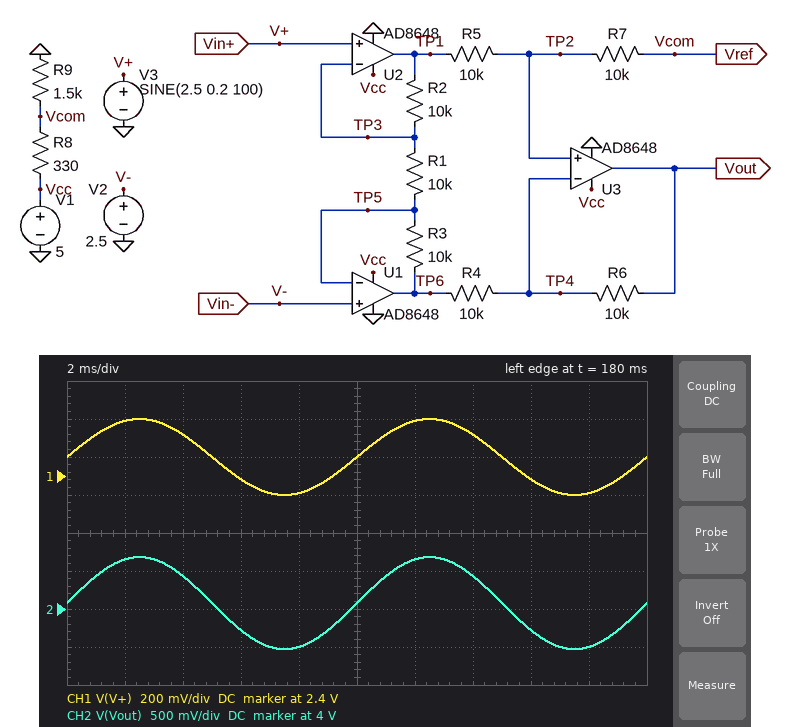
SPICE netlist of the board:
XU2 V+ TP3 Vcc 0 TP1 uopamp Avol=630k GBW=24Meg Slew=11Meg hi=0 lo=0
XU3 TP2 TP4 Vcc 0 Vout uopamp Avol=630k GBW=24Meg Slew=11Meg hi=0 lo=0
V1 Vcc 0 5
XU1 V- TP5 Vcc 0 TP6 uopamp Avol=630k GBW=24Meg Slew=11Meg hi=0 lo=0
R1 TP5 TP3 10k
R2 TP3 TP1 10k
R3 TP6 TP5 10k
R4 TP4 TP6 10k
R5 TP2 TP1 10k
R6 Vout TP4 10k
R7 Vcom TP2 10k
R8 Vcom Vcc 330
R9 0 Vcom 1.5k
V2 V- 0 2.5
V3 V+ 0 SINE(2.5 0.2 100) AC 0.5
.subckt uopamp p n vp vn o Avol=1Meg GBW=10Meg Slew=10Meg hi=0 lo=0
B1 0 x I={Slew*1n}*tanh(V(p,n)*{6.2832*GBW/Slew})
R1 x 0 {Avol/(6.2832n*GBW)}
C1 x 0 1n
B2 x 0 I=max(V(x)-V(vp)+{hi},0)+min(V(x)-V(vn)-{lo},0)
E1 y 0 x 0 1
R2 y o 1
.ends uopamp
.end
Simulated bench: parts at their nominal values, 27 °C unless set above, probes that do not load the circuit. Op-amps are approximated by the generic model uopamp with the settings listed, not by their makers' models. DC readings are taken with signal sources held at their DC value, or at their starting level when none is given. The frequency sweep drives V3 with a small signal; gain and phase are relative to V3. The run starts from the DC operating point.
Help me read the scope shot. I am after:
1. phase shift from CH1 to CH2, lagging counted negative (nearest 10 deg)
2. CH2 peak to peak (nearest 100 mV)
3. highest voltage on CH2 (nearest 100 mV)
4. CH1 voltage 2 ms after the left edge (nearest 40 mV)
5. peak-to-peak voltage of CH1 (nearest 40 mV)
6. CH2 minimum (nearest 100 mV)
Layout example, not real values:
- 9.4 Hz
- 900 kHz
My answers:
- 0 deg
- 1.2 V
- 4.7 V
- 2.68 V
- 400 mV
- 3.5 V
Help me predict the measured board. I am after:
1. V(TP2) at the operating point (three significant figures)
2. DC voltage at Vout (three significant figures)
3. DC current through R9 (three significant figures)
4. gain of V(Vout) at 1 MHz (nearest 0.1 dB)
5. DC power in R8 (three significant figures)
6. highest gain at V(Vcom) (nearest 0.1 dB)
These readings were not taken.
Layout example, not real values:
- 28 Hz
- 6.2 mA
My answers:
- 3.29 V
- 4.08 V
- 2.72 mA
- 9.5 dB
- 2.58 mW
- -31.5 dB
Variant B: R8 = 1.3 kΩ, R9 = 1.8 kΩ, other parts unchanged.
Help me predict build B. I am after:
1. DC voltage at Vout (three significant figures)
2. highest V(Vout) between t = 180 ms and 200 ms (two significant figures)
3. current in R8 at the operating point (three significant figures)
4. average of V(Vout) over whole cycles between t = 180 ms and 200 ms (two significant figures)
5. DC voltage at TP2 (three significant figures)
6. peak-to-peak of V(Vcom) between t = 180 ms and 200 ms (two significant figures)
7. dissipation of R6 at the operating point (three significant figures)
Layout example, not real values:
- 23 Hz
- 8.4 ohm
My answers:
- 2.89 V
- 3.5 V
- 1.62 mA
- 2.9 V
- 2.69 V
- 29 mV
- 3.77 µW
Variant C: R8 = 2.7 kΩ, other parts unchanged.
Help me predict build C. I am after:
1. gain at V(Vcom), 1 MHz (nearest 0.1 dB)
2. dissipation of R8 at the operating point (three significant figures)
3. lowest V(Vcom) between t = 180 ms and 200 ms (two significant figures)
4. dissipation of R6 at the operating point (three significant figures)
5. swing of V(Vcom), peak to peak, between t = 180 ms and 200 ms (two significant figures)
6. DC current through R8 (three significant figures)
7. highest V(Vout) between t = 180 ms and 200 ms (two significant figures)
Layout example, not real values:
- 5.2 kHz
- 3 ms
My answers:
- -20.8 dB
- 3.75 mW
- 1.8 V
- 11.6 µW
- 37 mV
- 1.18 mA
- 2.4 V
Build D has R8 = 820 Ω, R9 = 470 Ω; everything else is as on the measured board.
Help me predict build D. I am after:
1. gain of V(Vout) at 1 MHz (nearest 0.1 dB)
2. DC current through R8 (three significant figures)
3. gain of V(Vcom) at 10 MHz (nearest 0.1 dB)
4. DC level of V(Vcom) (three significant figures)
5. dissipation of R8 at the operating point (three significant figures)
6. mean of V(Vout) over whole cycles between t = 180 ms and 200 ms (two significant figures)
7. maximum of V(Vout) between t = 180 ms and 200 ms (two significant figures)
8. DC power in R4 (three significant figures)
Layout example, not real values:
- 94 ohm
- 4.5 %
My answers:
- 9.5 dB
- 3.86 mA
- -34.0 dB
- 1.83 V
- 12.2 mW
- 1.8 V
- 2.4 V
- 11.2 µW
